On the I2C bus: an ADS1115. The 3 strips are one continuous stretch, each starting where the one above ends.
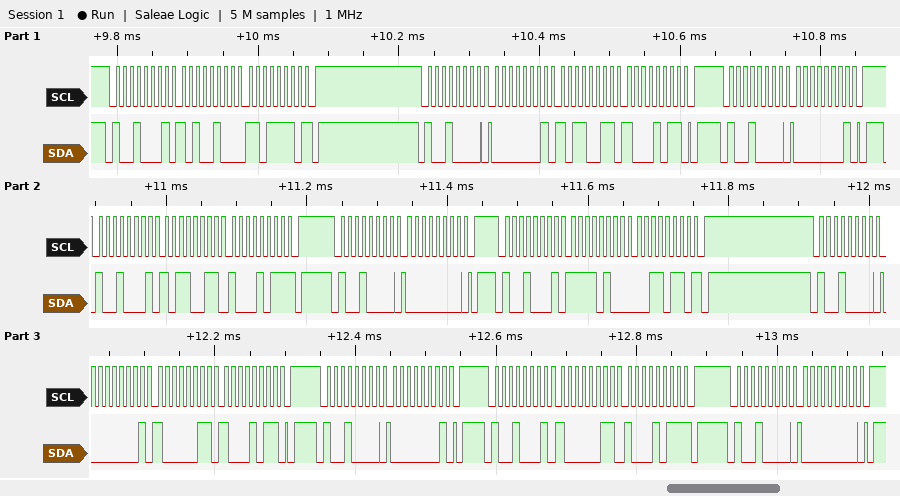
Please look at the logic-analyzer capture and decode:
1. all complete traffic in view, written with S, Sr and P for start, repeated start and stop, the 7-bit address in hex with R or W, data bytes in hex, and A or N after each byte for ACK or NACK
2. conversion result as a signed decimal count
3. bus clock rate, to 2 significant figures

S 48R A A4 A DE N P S 48W A 01 A B3 A 8B A P S 48W A 01 A P S 48R A B3 A 8B N P S 48W A 00 A P S 48R A F4 A 36 N P S 48W A 01 A 83 A 8B A P S 48W A 01 A P S 48R A 83 A 8B N P S 48W A 00 A P
-3018
100 kHz
